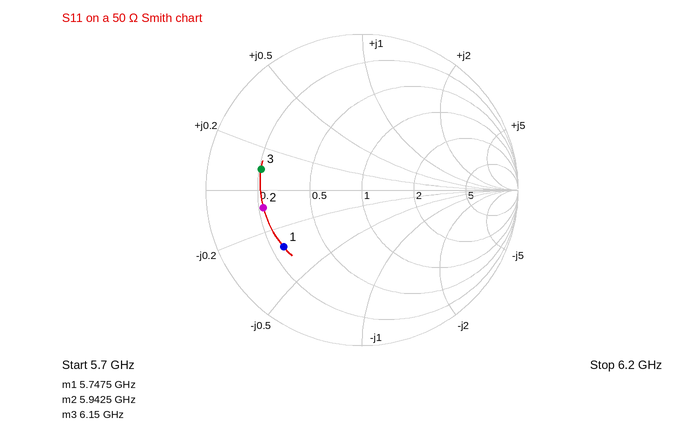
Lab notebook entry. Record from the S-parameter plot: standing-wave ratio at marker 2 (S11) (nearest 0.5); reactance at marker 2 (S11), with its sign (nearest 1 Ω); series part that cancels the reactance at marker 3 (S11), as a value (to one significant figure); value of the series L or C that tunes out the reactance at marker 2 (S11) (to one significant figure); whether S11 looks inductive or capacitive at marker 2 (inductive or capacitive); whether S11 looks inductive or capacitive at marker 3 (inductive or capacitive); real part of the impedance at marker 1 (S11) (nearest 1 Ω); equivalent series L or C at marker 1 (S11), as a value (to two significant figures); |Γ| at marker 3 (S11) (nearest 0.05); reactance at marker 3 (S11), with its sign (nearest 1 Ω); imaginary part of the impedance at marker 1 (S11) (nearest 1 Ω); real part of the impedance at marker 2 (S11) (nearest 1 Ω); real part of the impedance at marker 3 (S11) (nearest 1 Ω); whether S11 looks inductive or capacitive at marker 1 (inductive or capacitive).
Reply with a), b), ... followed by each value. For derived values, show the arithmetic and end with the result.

a) 4.5
b) -4 Ω
c) C = 1/(2π × 6.15 GHz × 5 Ω) ≈ 5 pF
d) L = 4 Ω/(2π × 5.9425 GHz) ≈ 107 pH, so 100 pH to one significant figure
e) capacitive
f) inductive
g) 13 Ω
h) C = 1/(2π × 5.7475 GHz × 15 Ω) ≈ 1.8 pF
i) 0.65
j) +5 Ω
k) -15 Ω
l) 11 Ω
m) 10 Ω
n) capacitive
